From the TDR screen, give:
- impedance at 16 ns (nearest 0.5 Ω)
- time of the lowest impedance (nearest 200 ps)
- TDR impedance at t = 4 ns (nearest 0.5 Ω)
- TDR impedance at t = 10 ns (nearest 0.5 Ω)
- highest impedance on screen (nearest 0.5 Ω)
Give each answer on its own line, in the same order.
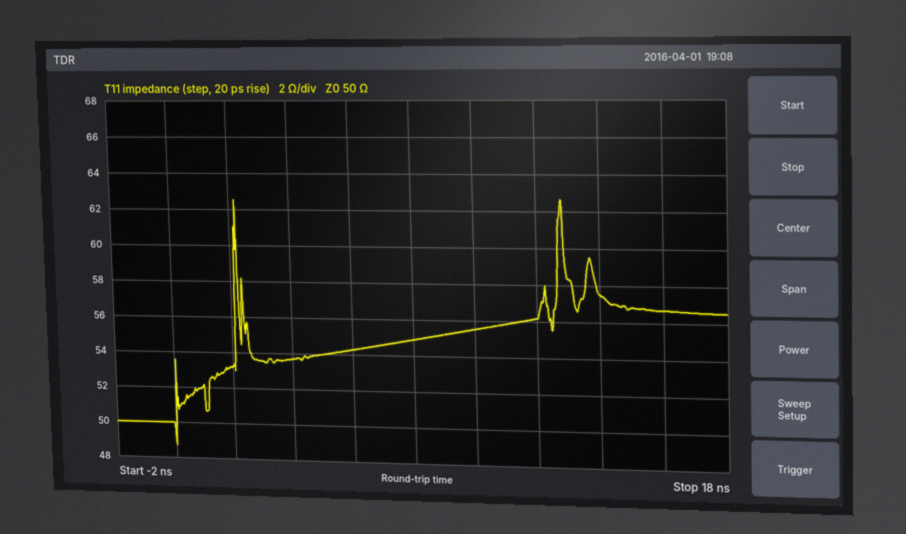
56.5 Ω
0.0 ns
53.5 Ω
55.5 Ω
62.5 Ω
